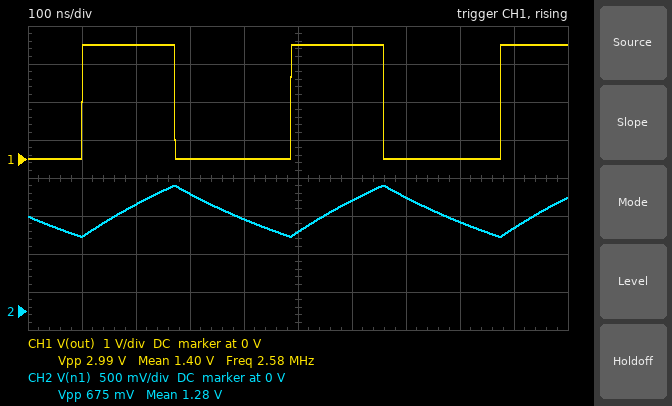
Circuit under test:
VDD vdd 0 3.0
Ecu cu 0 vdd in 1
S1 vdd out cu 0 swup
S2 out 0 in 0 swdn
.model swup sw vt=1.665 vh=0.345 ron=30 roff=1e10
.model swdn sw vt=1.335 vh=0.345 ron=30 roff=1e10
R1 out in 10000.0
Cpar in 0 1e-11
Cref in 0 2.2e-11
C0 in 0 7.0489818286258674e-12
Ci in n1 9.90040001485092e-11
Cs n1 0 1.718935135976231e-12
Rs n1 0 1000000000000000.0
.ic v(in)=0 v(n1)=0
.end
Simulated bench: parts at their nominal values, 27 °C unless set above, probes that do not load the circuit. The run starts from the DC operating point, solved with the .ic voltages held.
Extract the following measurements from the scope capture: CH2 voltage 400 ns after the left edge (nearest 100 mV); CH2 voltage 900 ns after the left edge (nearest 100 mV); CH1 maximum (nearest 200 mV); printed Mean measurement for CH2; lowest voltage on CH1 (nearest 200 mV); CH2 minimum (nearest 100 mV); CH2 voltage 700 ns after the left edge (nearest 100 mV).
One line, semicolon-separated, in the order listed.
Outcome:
1.2 V; 1.1 V; 3.0 V; 1.28 V; 0 V; 1.0 V; 1.5 V
